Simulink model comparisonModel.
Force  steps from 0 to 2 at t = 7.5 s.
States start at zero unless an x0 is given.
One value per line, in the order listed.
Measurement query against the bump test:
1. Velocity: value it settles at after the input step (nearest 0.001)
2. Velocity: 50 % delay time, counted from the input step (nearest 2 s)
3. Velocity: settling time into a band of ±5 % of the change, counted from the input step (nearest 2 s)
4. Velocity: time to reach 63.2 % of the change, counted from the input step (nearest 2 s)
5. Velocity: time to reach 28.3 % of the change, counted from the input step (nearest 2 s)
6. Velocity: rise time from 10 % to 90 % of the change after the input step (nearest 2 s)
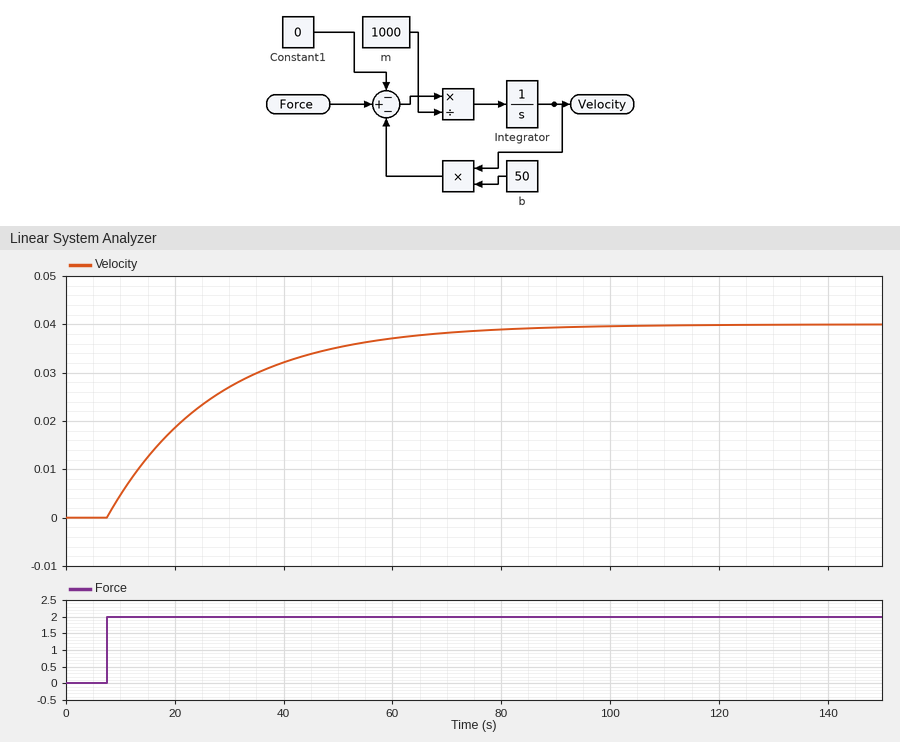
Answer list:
0.040
14 s
60 s
20 s
6 s
44 s
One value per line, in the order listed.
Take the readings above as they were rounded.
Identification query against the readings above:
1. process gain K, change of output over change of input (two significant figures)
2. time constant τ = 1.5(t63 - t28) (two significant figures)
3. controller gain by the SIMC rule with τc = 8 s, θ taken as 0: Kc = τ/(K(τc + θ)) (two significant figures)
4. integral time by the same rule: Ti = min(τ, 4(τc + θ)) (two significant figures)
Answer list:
0.020
21 s
130
21 s
